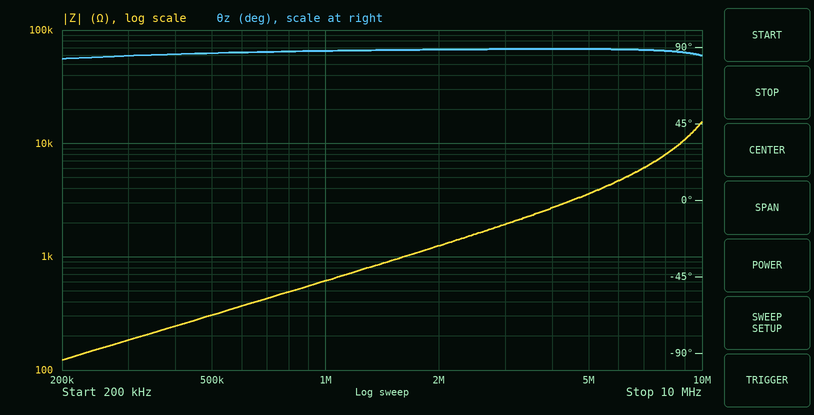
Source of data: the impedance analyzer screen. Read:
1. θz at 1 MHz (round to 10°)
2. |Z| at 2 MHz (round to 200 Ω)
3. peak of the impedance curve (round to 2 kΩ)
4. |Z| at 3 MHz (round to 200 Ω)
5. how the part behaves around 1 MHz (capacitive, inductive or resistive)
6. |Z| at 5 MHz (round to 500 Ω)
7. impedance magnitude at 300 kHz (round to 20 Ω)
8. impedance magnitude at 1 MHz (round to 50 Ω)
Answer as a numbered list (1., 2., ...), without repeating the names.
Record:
1. 90°
2. 1.2 kΩ
3. 16 kΩ
4. 2.0 kΩ
5. inductive
6. 3.5 kΩ
7. 180 Ω
8. 600 Ω
